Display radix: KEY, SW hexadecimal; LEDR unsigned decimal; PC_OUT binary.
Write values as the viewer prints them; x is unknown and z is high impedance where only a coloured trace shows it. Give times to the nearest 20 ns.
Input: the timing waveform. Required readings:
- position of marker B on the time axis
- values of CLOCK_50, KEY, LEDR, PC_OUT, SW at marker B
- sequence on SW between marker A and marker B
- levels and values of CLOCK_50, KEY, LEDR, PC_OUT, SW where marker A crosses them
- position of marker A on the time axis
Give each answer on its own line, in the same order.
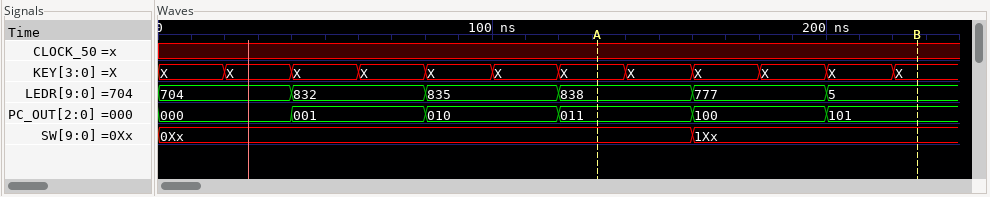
220 ns
CLOCK_50=x, KEY=X, LEDR=5, PC_OUT=101, SW=1Xx
0Xx, 1Xx
CLOCK_50=x, KEY=X, LEDR=838, PC_OUT=011, SW=0Xx
140 ns
